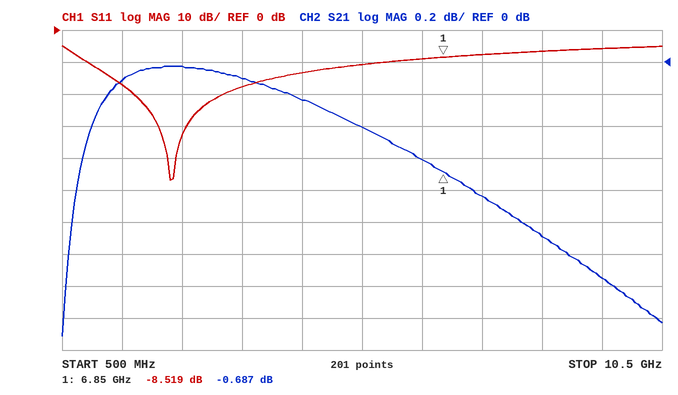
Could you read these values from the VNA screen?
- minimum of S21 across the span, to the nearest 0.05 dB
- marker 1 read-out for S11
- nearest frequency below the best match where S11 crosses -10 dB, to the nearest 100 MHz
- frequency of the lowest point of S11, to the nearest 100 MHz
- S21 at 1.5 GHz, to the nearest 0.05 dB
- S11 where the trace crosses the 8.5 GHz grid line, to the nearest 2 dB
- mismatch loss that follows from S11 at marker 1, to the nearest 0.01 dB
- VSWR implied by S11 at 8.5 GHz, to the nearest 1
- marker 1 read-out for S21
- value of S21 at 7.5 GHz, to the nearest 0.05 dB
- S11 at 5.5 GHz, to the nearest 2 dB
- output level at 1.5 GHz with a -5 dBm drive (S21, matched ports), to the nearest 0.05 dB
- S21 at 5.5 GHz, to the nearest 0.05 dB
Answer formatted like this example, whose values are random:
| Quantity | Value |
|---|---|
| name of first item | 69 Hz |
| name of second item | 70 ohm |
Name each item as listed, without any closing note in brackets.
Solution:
| Quantity | Value |
|---|---|
| minimum of S21 across the span, to the nearest 0.05 dB | -1.70 dB |
| marker 1 read-out for S11 | -8.519 dB |
| nearest frequency below the best match where S11 crosses -10 dB, to the nearest 100 MHz | 900 MHz |
| frequency of the lowest point of S11, to the nearest 100 MHz | 2.3 GHz |
| S21 at 1.5 GHz, to the nearest 0.05 dB | -0.10 dB |
| S11 where the trace crosses the 8.5 GHz grid line, to the nearest 2 dB | -6 dB |
| mismatch loss that follows from S11 at marker 1, to the nearest 0.01 dB | 0.66 dB |
| VSWR implied by S11 at 8.5 GHz, to the nearest 1 | 3 |
| marker 1 read-out for S21 | -0.687 dB |
| value of S21 at 7.5 GHz, to the nearest 0.05 dB | -0.85 dB |
| S11 at 5.5 GHz, to the nearest 2 dB | -10 dB |
| output level at 1.5 GHz with a -5 dBm drive (S21, matched ports), to the nearest 0.05 dB | -5.10 dBm |
| S21 at 5.5 GHz, to the nearest 0.05 dB | -0.40 dB |
